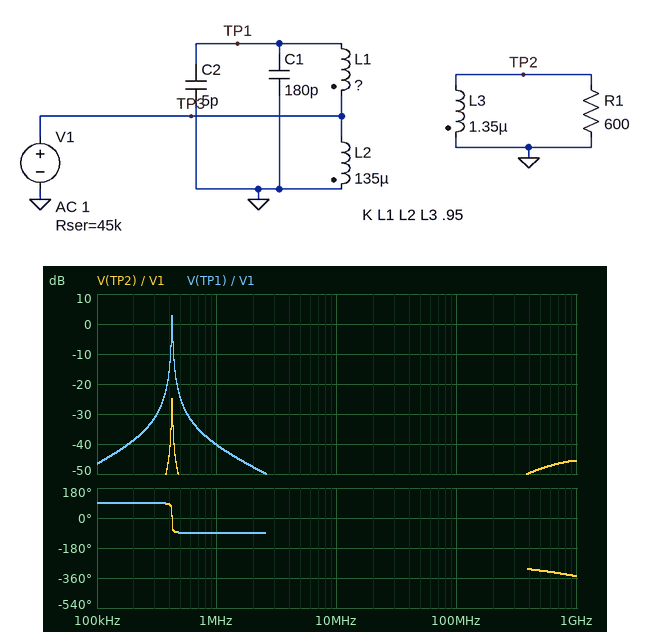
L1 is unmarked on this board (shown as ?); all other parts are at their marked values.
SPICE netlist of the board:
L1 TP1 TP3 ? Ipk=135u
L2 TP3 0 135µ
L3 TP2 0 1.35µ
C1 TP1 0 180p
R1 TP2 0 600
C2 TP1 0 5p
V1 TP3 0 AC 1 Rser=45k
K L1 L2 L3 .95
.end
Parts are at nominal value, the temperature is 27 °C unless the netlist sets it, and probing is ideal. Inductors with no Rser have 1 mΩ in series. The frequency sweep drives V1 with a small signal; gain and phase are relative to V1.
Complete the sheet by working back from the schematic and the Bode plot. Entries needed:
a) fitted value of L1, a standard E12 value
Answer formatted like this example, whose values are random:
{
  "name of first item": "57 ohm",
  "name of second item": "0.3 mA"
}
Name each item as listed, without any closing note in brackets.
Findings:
{
  "fitted value of L1, a standard E12 value": "270 µH"
}
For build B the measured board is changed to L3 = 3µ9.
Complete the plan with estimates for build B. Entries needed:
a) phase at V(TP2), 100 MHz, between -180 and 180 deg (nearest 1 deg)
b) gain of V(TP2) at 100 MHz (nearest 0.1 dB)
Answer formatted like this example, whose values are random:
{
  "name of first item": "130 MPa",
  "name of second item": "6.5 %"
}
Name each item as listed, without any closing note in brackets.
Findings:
{
  "phase at V(TP2), 100 MHz, between -180 and 180 deg": "69 deg",
  "gain of V(TP2) at 100 MHz": "-56.5 dB"
}
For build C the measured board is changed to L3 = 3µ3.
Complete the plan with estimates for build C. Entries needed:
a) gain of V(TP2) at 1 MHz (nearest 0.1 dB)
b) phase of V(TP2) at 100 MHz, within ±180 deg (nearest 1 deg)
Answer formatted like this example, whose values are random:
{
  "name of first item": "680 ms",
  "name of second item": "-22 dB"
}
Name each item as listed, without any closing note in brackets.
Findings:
{
  "gain of V(TP2) at 1 MHz": "-64.6 dB",
  "phase of V(TP2) at 100 MHz, within ±180 deg": "72 deg"
}
